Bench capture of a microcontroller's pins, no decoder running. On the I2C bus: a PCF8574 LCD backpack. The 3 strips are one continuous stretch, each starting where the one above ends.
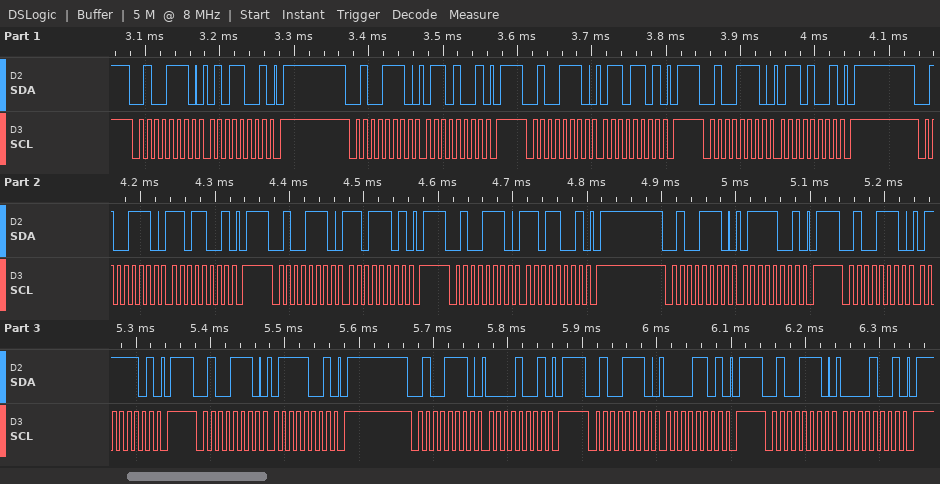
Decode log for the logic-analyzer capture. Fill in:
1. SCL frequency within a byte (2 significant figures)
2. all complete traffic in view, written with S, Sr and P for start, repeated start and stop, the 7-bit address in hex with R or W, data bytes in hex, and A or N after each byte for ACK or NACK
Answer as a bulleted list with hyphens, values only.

- 100 kHz
- S 27W A 59 A P S 27W A 69 A P S 27W A 6D A P S 27W A 69 A P S 27W A D9 A P S 27W A DD A P S 27W A D9 A P S 27W A 79 A P S 27W A 7D A P S 27W A 79 A P S 27W A 09 A P S 27W A 0D A P S 27W A 09 A P
